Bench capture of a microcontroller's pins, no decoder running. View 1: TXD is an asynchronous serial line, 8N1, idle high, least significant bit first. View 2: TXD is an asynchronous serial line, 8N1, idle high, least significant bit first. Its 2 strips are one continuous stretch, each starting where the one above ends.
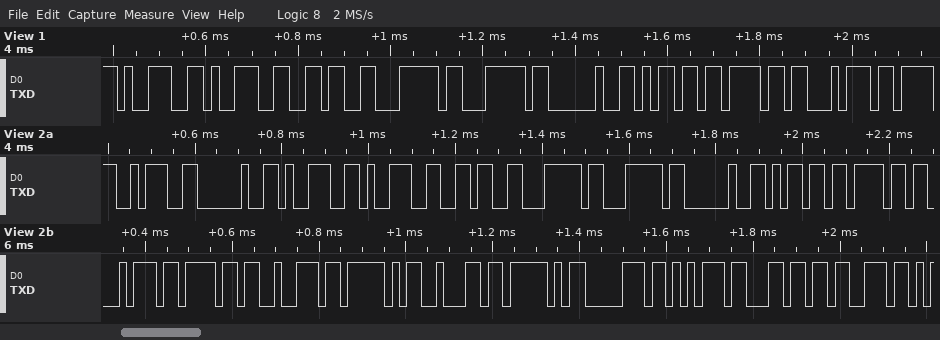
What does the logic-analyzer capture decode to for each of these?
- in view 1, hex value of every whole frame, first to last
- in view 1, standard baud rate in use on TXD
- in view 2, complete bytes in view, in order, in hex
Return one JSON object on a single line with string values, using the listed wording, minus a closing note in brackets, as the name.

{"in view 1, hex value of every whole frame, first to last": "39 39 36 7C 7C 20 6D 6F 74", "in view 1, standard baud rate in use on TXD": "57600 baud", "in view 2, complete bytes in view, in order, in hex": "3A 20 39 39 36 7C 7C 20 6D 6F 74 6F 72 5F 62 5F 70 75 6C 73"}
